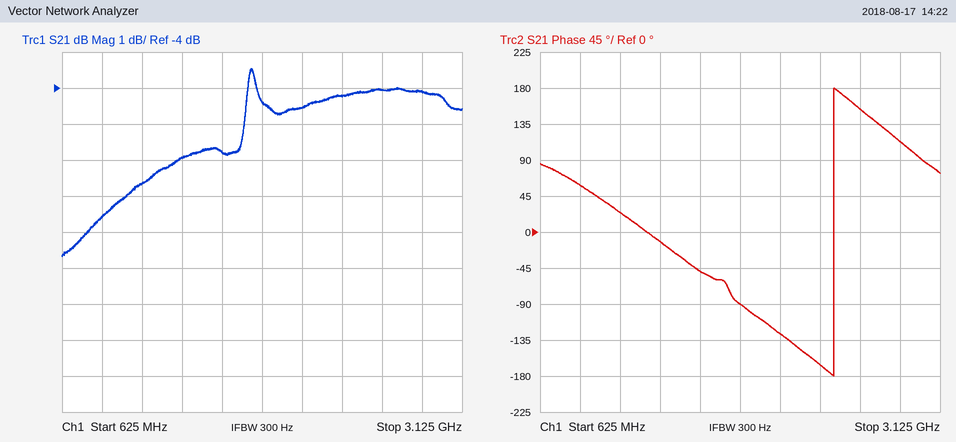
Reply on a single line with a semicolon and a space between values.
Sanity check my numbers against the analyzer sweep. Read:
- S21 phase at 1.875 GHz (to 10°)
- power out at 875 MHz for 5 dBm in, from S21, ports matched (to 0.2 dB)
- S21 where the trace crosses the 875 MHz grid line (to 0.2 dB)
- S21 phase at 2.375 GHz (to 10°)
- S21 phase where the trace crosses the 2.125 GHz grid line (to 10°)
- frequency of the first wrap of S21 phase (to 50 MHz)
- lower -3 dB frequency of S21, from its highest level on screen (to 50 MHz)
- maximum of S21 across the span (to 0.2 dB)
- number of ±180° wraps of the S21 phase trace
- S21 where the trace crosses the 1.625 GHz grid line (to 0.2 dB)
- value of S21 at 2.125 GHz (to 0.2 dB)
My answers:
-90°; -2.6 dBm; -7.6 dB; -170°; -130°; 2.45 GHz; 1.20 GHz; -3.4 dB; 1; -5.8 dB; -4.6 dB
